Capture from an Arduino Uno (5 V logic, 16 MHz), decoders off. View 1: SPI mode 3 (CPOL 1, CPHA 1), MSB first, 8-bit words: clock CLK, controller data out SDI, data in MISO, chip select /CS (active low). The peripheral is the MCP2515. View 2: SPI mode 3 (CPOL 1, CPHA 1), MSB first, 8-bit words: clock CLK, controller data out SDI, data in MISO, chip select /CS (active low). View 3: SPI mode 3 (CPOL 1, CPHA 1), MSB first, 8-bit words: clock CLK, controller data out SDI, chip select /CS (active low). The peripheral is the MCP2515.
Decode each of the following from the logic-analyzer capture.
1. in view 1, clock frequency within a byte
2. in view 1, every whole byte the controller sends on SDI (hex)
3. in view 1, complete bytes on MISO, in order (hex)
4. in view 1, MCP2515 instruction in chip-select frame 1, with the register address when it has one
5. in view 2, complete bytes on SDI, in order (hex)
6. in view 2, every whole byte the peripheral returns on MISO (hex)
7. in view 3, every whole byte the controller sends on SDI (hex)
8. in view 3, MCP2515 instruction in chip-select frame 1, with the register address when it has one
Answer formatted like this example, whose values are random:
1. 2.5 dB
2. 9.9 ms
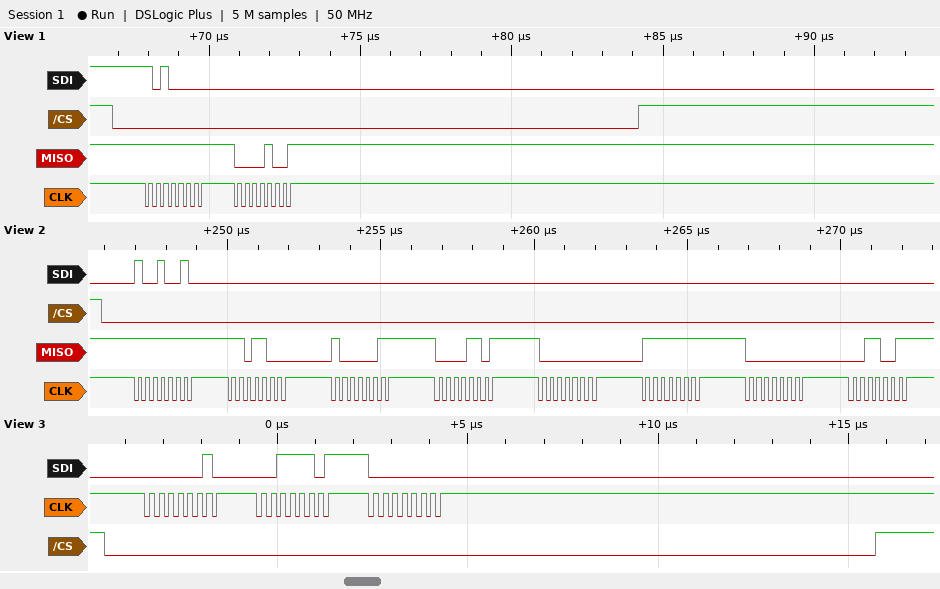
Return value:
1. 4 MHz
2. 0xA0 0x00
3. 0xFF 0x09
4. READ STATUS
5. 0x92 0x00 0x00 0x00 0x00 0x00 0x00 0x00
6. 0xFF 0xD8 0x83 0x0D 0x00 0xFF 0x00 0x33
7. 02 3D 00
8. WRITE 0x3D
